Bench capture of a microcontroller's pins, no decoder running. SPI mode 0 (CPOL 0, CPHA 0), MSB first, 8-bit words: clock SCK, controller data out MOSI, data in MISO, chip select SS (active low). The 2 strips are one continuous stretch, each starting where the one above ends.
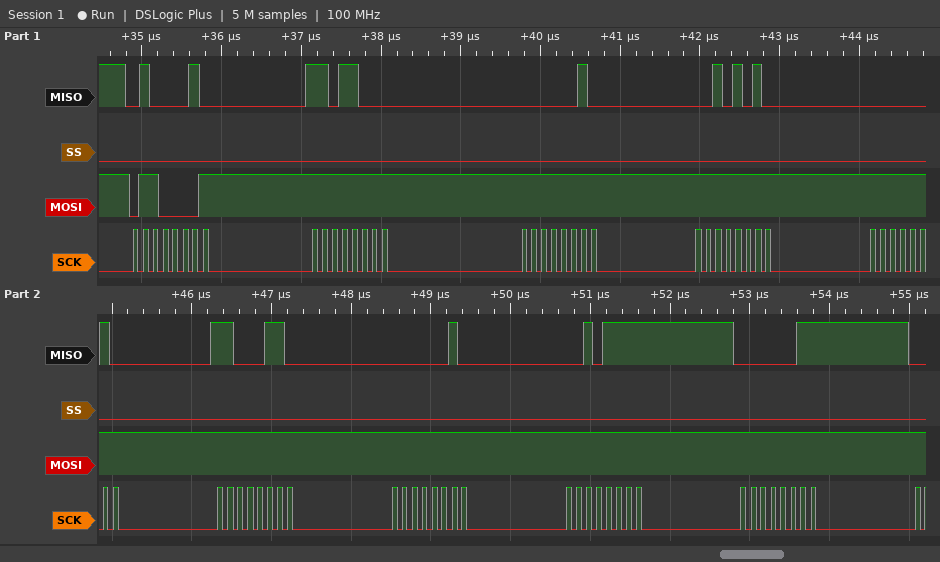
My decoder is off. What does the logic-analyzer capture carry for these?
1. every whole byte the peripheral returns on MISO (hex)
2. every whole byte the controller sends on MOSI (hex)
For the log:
42 D8 02 2A 02 C6 02 2F 03
61 FF FF FF FF FF FF FF FF
